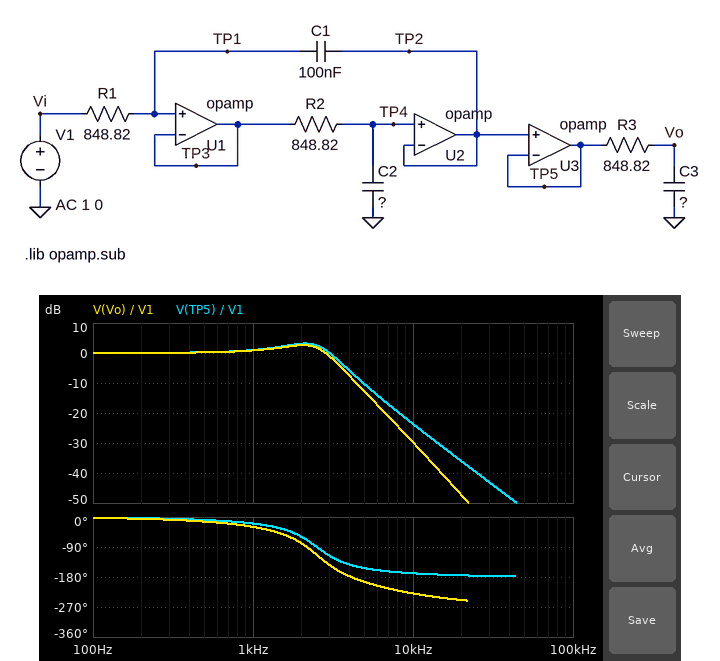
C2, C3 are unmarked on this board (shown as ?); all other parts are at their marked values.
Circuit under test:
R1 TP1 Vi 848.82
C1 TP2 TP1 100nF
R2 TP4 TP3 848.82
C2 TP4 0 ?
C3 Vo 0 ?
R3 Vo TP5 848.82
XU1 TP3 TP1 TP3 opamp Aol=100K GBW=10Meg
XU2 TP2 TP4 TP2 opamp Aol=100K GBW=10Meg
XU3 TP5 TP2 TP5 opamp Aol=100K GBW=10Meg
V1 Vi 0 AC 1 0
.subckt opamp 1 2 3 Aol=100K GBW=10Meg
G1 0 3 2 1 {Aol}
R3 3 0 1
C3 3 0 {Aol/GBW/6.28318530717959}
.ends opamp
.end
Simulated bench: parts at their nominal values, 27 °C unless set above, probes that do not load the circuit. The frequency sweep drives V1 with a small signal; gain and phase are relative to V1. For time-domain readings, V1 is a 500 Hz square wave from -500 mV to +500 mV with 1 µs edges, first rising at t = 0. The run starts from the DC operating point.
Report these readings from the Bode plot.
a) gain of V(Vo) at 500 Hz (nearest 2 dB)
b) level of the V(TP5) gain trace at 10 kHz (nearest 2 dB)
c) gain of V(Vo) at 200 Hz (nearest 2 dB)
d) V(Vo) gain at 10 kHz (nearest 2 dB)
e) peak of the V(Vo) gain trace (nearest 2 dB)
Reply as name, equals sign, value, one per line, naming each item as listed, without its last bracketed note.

gain of V(Vo) at 500 Hz = 0 dB
level of the V(TP5) gain trace at 10 kHz = -24 dB
gain of V(Vo) at 200 Hz = 0 dB
V(Vo) gain at 10 kHz = -30 dB
peak of the V(Vo) gain trace = 2 dB
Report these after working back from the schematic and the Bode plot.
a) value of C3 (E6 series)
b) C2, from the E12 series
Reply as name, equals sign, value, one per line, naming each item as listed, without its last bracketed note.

value of C3 = 33 nF
C2, from the E12 series = 56 nF
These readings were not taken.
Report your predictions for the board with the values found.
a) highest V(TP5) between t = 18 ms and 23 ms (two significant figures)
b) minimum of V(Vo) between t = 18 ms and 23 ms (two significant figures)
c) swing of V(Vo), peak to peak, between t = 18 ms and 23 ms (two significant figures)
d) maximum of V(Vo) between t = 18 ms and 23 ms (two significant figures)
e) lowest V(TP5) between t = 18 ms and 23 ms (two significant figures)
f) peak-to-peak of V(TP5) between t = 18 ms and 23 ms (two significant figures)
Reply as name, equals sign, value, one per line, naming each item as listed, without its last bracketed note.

highest V(TP5) between t = 18 ms and 23 ms = 780 mV
minimum of V(Vo) between t = 18 ms and 23 ms = -750 mV
swing of V(Vo), peak to peak, between t = 18 ms and 23 ms = 1.5 V
maximum of V(Vo) between t = 18 ms and 23 ms = 750 mV
lowest V(TP5) between t = 18 ms and 23 ms = -780 mV
peak-to-peak of V(TP5) between t = 18 ms and 23 ms = 1.6 V
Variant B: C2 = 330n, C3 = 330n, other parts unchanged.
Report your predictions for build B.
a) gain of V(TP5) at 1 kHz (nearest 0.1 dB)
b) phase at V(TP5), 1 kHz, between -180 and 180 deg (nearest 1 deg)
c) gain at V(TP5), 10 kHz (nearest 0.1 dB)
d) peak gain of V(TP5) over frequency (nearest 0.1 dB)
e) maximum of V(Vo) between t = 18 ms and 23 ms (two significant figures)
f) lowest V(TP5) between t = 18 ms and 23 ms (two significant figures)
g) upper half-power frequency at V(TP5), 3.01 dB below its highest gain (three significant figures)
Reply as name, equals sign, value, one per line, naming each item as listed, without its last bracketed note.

gain of V(TP5) at 1 kHz = -4.9 dB
phase at V(TP5), 1 kHz, between -180 and 180 deg = -88 deg
gain at V(TP5), 10 kHz = -39.5 dB
peak gain of V(TP5) over frequency = 0 dB
maximum of V(Vo) between t = 18 ms and 23 ms = 420 mV
lowest V(TP5) between t = 18 ms and 23 ms = -500 mV
upper half-power frequency at V(TP5), 3.01 dB below its highest gain = 760 Hz
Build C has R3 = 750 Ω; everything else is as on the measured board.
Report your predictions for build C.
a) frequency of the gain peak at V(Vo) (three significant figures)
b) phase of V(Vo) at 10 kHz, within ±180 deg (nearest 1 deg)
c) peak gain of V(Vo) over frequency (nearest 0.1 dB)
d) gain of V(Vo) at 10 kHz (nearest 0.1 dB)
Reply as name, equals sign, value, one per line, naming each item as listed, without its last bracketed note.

frequency of the gain peak at V(Vo) = 2.08 kHz
phase of V(Vo) at 10 kHz, within ±180 deg = 134 deg
peak gain of V(Vo) over frequency = 2.7 dB
gain of V(Vo) at 10 kHz = -29.0 dB
